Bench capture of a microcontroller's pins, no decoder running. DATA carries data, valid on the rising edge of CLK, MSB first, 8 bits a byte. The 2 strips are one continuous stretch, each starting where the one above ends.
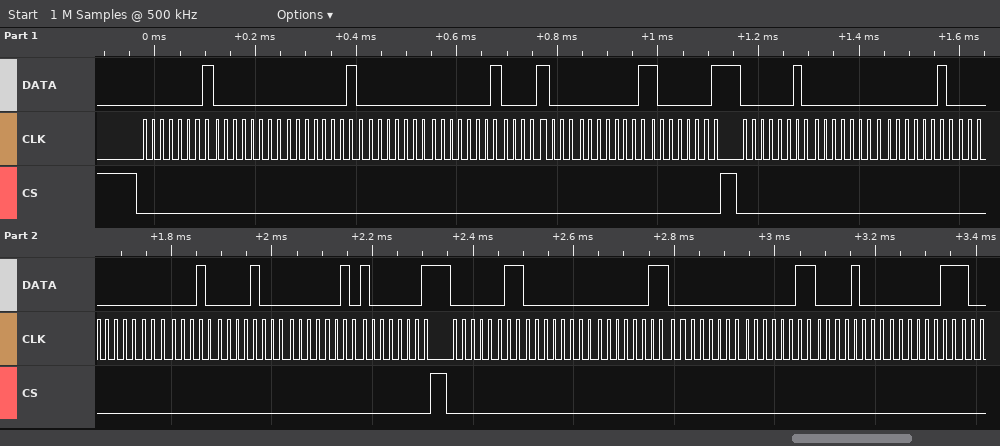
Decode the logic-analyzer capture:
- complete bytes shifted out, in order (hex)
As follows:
01 00 01 00 01 08 01 81 02 00 02 00 02 08 02 81 03 00 03 00 03 08 03
